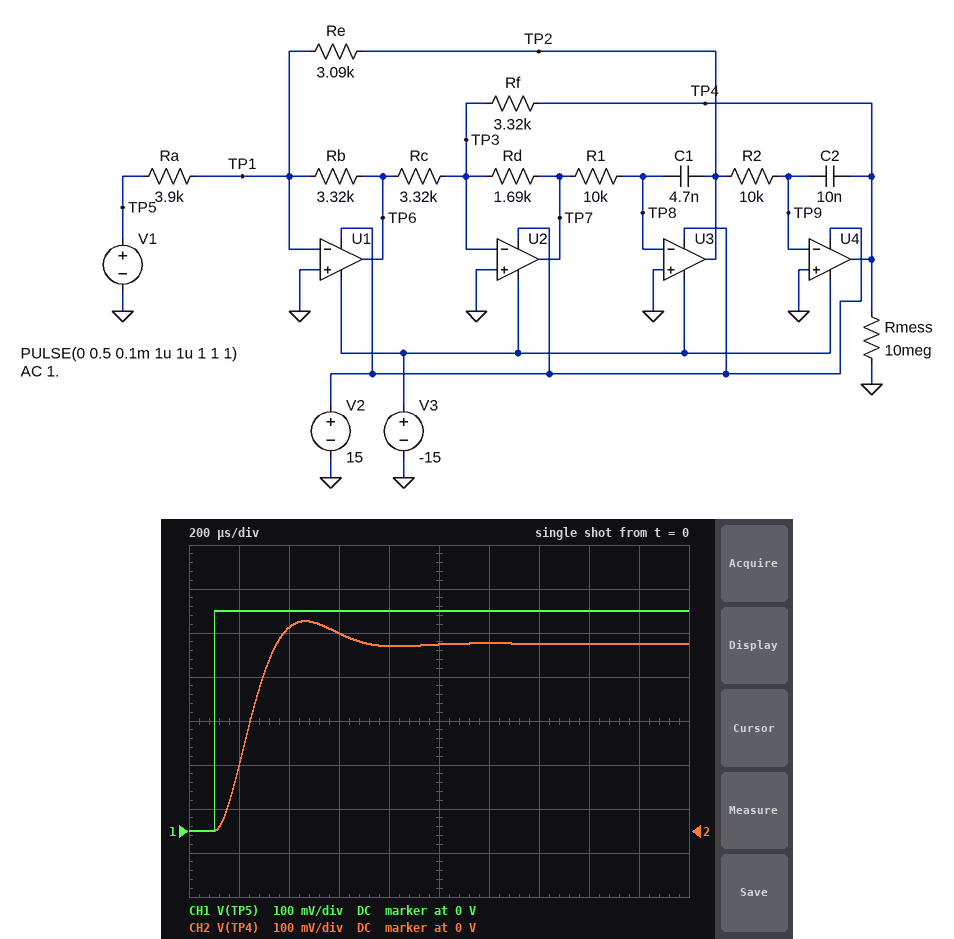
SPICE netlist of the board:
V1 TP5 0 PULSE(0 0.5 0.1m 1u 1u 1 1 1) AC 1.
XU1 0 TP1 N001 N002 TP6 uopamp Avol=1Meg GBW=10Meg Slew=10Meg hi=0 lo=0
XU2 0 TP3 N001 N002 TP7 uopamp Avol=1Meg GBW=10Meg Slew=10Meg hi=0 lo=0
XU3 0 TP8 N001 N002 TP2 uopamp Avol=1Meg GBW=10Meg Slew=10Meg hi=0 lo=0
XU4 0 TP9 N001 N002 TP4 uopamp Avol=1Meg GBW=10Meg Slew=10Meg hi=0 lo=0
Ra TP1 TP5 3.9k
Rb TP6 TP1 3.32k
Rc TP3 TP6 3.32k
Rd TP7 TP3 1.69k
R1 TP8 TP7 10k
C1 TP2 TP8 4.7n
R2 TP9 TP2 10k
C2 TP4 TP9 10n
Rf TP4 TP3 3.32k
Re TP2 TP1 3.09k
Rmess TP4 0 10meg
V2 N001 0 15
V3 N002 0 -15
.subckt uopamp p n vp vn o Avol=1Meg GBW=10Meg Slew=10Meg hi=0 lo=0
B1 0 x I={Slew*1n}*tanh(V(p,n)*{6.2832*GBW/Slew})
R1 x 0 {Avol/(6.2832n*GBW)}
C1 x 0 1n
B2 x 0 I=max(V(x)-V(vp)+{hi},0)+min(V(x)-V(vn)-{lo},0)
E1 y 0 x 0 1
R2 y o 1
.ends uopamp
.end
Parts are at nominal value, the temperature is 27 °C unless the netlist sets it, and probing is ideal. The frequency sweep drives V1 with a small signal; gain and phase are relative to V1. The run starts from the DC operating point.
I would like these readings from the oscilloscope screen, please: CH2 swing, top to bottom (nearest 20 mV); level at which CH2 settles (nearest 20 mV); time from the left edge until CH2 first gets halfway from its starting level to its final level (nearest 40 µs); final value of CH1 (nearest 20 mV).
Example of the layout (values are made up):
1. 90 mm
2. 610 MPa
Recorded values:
1. 480 mV
2. 420 mV
3. 240 µs
4. 500 mV
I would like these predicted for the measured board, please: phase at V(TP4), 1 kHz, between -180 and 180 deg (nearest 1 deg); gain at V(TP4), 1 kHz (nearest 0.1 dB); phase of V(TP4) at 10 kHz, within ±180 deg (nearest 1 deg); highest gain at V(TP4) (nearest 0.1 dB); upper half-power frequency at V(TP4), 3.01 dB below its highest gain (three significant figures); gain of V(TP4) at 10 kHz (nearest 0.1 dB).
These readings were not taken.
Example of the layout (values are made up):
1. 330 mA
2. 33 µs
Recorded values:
1. -47 deg
2. -0.7 dB
3. -170 deg
4. -0.7 dB
5. 1.89 kHz
6. -32.5 dB
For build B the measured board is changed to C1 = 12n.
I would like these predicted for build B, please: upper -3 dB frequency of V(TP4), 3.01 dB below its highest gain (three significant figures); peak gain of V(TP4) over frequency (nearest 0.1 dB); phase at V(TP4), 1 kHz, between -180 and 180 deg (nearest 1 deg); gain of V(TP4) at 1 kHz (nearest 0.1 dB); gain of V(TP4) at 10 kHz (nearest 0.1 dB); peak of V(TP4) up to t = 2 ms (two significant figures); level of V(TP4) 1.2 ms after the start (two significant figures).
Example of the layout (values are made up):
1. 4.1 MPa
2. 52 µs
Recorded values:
1. 1.23 kHz
2. 2.3 dB
3. -84 deg
4. 2.0 dB
5. -40.7 dB
6. 560 mV
7. 390 mV
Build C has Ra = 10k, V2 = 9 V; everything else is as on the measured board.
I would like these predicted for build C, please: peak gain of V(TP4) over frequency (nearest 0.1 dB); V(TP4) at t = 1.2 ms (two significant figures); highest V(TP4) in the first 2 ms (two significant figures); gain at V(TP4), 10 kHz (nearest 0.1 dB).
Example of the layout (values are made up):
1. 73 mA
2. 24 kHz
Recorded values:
1. -8.9 dB
2. 170 mV
3. 190 mV
4. -40.7 dB
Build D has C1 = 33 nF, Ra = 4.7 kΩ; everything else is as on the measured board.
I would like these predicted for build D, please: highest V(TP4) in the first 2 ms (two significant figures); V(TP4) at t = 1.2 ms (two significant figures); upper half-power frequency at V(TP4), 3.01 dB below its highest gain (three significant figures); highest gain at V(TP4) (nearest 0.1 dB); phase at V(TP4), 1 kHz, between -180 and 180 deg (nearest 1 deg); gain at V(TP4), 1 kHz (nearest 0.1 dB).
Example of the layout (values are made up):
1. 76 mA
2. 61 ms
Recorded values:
1. 530 mV
2. 450 mV
3. 719 Hz
4. 4.7 dB
5. -157 deg
6. -7.6 dB
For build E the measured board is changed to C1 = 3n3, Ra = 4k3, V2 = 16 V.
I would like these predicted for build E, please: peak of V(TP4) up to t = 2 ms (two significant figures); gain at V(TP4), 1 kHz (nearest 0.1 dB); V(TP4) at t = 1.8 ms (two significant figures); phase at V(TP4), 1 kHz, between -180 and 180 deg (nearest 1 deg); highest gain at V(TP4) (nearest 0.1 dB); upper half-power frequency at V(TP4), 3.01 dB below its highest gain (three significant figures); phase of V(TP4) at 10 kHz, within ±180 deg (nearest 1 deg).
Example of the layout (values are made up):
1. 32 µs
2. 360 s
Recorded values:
1. 410 mV
2. -2.3 dB
3. 390 mV
4. -42 deg
5. -2.2 dB
6. 2.08 kHz
7. -165 deg
